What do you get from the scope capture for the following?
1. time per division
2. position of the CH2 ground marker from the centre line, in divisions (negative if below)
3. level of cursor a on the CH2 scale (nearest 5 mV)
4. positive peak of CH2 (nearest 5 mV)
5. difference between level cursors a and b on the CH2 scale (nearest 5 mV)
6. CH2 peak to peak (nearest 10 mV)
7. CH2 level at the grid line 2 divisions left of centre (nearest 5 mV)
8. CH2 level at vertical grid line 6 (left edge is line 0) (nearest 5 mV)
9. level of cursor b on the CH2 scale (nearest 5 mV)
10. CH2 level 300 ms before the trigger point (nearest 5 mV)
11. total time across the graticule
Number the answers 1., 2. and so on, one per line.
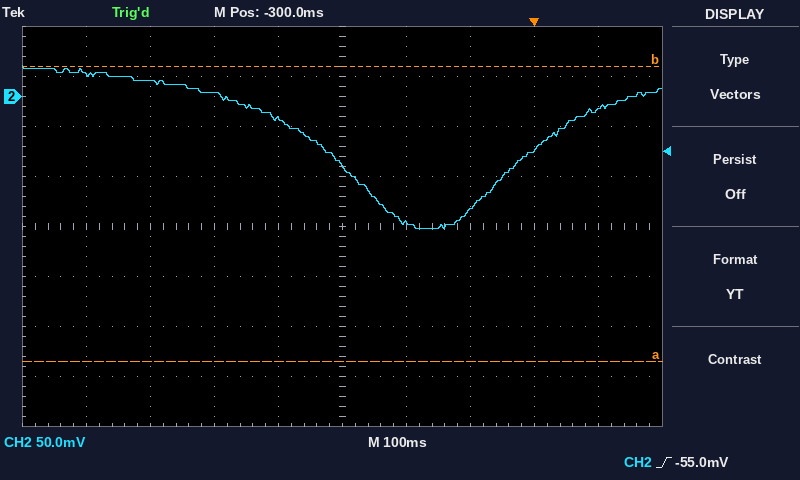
1. 100 ms
2. +2.6 div
3. -265 mV
4. 30 mV
5. 295 mV
6. 160 mV
7. 5 mV
8. -125 mV
9. 30 mV
10. -70 mV
11. 1 s
